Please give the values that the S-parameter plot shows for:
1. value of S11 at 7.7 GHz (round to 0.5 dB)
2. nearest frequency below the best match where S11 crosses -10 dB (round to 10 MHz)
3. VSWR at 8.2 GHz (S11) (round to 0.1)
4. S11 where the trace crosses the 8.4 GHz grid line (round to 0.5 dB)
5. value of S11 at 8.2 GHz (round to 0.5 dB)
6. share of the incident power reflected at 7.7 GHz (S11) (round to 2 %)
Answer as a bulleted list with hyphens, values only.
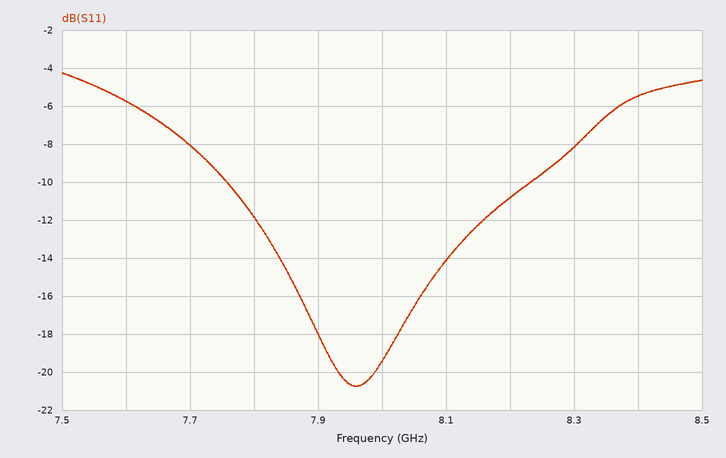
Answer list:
- -8.0 dB
- 7.76 GHz
- 1.8
- -5.5 dB
- -11.0 dB
- 16 %
